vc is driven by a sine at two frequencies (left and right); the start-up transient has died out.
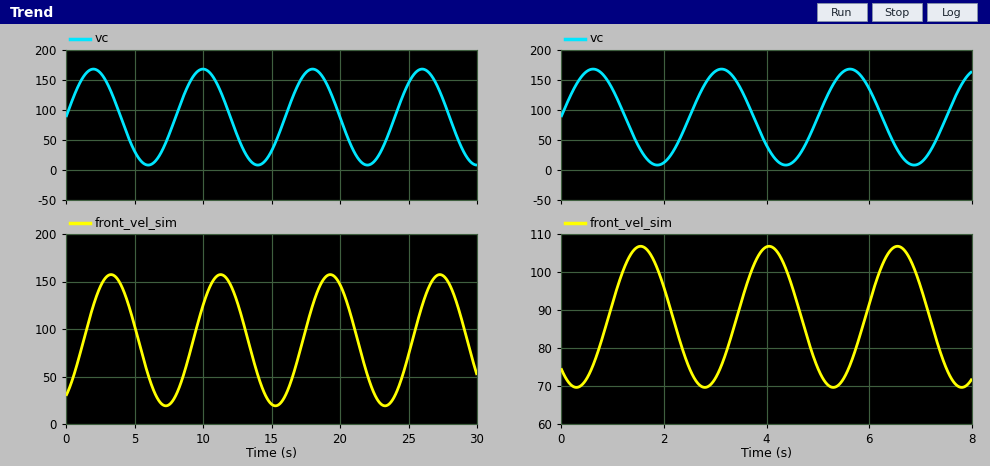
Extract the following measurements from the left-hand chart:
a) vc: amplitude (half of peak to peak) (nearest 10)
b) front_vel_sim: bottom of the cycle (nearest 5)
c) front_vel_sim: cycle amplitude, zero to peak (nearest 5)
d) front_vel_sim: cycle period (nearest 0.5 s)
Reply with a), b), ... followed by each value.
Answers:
a) 80
b) 20
c) 70
d) 8.0 s
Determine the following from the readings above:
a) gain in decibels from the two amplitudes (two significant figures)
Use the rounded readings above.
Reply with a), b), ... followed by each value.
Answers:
a) -1.2 dB
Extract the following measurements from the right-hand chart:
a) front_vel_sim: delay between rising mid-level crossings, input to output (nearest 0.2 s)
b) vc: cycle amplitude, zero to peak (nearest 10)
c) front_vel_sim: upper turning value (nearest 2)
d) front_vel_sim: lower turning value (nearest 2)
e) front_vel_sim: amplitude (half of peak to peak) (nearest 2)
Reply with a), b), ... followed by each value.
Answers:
a) 1.0 s
b) 80
c) 106
d) 70
e) 18
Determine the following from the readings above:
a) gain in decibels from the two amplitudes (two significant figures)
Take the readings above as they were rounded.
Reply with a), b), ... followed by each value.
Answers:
a) -13 dB
